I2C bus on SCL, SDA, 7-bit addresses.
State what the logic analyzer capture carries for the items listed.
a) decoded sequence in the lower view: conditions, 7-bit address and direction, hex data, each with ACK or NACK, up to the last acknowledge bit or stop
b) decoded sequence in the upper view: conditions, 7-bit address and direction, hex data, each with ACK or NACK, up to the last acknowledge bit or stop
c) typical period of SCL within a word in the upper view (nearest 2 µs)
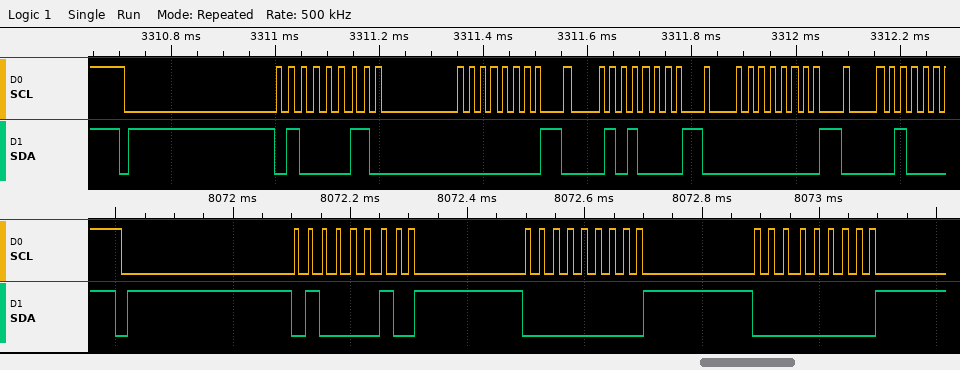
start, address 21 write ACK, 00 ACK, 00 ACK
start, address 21 read ACK, 00 ACK, 50 ACK, 00 ACK
22 µs
